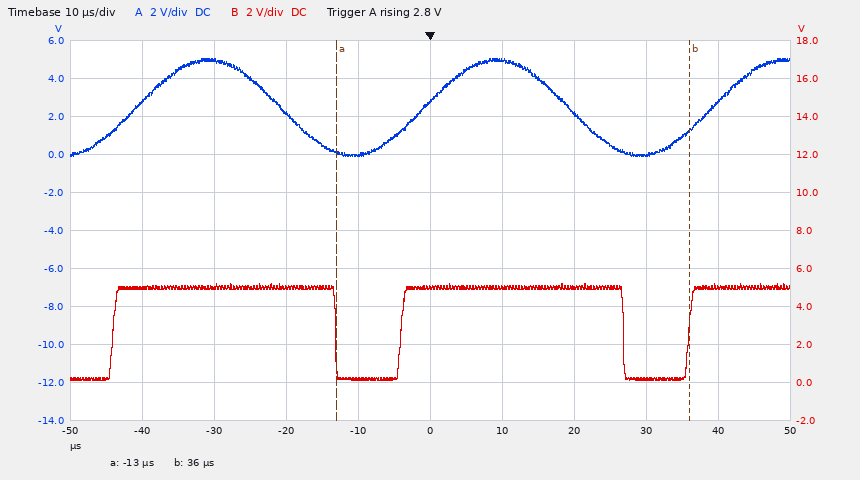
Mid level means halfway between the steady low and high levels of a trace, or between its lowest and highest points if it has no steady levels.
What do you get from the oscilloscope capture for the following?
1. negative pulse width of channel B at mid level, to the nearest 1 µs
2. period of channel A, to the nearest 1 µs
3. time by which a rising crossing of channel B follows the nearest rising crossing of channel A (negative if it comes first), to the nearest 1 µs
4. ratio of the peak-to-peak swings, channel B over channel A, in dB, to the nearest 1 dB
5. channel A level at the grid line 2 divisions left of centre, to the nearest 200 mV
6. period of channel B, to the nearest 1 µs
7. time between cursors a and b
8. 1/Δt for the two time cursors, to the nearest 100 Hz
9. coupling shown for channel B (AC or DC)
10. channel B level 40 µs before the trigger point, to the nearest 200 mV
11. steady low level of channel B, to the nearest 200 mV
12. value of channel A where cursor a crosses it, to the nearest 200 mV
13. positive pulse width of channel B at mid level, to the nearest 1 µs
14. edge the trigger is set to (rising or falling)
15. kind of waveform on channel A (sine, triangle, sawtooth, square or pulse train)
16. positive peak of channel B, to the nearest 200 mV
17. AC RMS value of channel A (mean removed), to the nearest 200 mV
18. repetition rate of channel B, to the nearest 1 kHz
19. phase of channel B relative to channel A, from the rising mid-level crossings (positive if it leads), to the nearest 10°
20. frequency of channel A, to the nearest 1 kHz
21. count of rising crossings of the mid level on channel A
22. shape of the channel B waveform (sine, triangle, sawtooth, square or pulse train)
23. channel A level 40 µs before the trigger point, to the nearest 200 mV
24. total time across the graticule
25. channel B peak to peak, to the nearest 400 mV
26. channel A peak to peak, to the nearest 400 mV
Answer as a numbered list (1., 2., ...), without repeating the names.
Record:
1. 9 µs
2. 40 µs
3. -3 µs
4. 0 dB
5. 2.2 V
6. 40 µs
7. 49 µs
8. 20.4 kHz
9. DC
10. 5.0 V
11. 200 mV
12. 200 mV
13. 31 µs
14. rising
15. sine
16. 5.2 V
17. 1.8 V
18. 25 kHz
19. +30°
20. 25 kHz
21. 3
22. pulse train
23. 2.8 V
24. 100 µs
25. 5.2 V
26. 5.2 V
